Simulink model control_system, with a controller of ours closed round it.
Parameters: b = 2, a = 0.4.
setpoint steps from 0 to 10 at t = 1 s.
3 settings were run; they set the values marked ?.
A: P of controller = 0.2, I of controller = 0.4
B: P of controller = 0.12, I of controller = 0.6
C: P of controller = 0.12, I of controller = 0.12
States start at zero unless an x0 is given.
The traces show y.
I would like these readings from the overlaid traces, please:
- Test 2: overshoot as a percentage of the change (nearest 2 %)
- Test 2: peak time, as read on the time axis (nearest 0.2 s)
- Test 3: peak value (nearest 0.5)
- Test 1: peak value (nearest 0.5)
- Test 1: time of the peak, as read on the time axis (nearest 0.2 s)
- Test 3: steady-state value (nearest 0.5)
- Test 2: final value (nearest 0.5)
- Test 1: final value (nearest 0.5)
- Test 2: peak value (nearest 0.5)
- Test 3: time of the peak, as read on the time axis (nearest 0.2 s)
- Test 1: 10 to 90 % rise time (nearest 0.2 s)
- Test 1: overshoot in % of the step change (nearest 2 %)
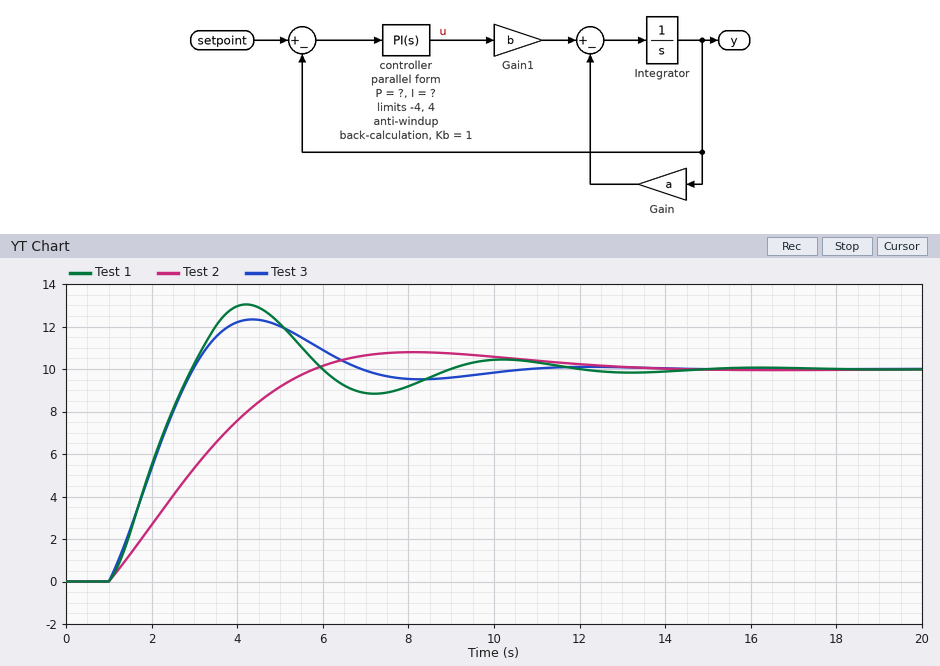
8 %
8.2 s
12.5
13.0
4.2 s
10.0
10.0
10.0
11.0
4.4 s
1.4 s
30 %
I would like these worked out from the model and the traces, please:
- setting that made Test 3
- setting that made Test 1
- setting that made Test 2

A
B
C
